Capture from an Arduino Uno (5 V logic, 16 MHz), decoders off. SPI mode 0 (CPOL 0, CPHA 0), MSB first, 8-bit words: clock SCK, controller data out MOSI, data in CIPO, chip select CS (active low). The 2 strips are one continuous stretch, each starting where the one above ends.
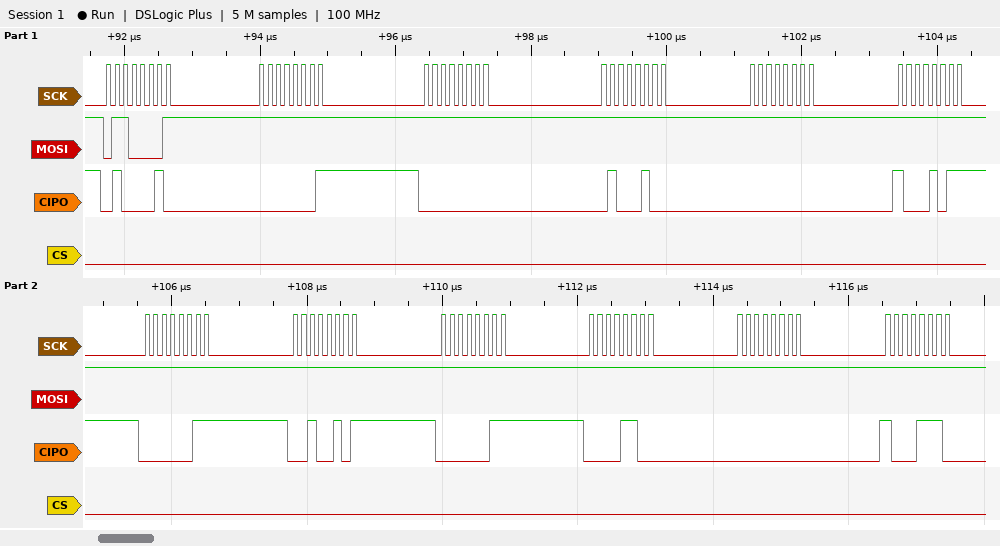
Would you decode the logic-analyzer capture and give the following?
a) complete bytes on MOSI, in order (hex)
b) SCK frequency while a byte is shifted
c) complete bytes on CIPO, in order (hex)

0x61 0xFF 0xFF 0xFF 0xFF 0xFF 0xFF 0xFF 0xFF 0xFF 0xFF 0xFF
8 MHz
0x42 0x01 0x00 0x44 0x00 0x8B 0x03 0x25 0x03 0x0C 0x00 0x8E
